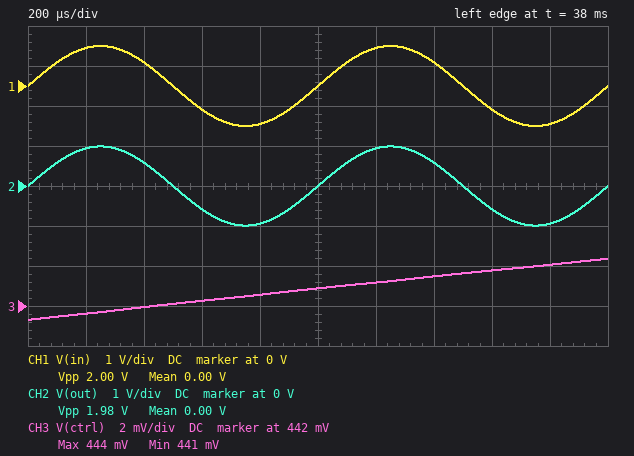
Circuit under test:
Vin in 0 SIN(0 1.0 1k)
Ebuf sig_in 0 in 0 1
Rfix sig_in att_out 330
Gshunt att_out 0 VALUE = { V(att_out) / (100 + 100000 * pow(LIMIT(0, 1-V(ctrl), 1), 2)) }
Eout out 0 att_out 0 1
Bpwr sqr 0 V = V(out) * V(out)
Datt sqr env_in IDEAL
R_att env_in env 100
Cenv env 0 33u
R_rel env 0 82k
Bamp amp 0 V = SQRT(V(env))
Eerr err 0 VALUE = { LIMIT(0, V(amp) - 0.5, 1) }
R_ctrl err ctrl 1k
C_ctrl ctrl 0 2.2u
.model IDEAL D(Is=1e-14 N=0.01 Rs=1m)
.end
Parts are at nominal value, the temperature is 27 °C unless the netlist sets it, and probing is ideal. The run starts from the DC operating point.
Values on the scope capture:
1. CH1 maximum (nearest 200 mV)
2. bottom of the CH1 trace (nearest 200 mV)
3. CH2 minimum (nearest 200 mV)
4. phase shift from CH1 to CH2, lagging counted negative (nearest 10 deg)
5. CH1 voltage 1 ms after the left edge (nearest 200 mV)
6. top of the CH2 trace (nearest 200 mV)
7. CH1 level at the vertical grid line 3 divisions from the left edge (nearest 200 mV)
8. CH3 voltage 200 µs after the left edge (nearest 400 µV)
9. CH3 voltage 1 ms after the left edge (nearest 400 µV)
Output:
1.0 V
-1.0 V
-1.0 V
0 deg
0 V
1.0 V
-600 mV
441.6 mV
442.8 mV
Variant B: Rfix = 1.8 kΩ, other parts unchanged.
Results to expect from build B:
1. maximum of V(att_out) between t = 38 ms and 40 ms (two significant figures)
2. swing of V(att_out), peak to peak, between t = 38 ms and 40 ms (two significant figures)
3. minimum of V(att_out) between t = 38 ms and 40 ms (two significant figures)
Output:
950 mV
1.9 V
-950 mV
